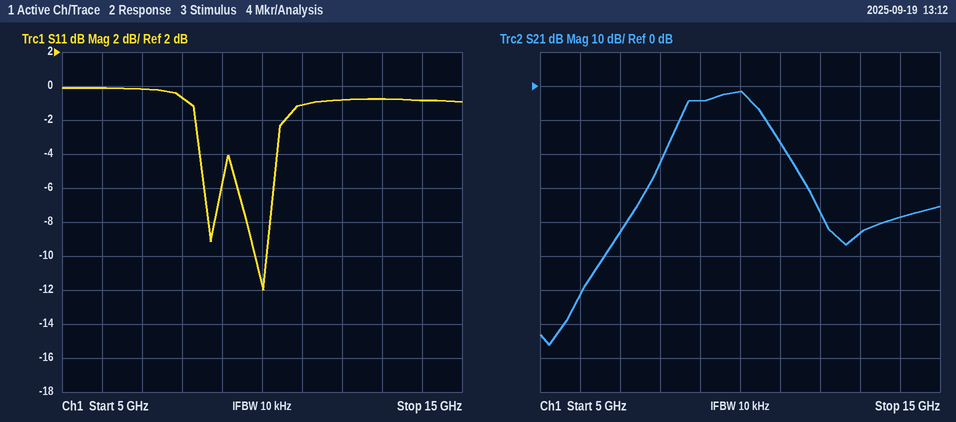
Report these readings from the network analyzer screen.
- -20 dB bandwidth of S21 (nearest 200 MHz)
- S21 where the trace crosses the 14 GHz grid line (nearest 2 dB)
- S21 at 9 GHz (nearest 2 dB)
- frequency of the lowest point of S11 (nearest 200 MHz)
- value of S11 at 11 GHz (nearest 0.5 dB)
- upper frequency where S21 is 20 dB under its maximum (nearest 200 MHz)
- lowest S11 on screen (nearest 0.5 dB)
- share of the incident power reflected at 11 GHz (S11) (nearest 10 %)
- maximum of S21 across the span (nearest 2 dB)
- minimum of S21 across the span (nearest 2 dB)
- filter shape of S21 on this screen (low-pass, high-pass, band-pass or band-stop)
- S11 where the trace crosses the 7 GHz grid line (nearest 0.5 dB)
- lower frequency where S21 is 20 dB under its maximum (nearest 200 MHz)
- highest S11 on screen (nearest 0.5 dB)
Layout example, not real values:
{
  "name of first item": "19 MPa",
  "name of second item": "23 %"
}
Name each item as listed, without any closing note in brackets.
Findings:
{
  "-20 dB bandwidth of S21": "3.2 GHz",
  "S21 where the trace crosses the 14 GHz grid line": "-38 dB",
  "S21 at 9 GHz": "-4 dB",
  "frequency of the lowest point of S11": "10.0 GHz",
  "value of S11 at 11 GHz": "-1.0 dB",
  "upper frequency where S21 is 20 dB under its maximum": "11.2 GHz",
  "lowest S11 on screen": "-12.0 dB",
  "share of the incident power reflected at 11 GHz (S11)": "80 %",
  "maximum of S21 across the span": "-2 dB",
  "minimum of S21 across the span": "-76 dB",
  "filter shape of S21 on this screen": "band-pass",
  "S11 where the trace crosses the 7 GHz grid line": "0.0 dB",
  "lower frequency where S21 is 20 dB under its maximum": "8.0 GHz",
  "highest S11 on screen": "0.0 dB"
}
